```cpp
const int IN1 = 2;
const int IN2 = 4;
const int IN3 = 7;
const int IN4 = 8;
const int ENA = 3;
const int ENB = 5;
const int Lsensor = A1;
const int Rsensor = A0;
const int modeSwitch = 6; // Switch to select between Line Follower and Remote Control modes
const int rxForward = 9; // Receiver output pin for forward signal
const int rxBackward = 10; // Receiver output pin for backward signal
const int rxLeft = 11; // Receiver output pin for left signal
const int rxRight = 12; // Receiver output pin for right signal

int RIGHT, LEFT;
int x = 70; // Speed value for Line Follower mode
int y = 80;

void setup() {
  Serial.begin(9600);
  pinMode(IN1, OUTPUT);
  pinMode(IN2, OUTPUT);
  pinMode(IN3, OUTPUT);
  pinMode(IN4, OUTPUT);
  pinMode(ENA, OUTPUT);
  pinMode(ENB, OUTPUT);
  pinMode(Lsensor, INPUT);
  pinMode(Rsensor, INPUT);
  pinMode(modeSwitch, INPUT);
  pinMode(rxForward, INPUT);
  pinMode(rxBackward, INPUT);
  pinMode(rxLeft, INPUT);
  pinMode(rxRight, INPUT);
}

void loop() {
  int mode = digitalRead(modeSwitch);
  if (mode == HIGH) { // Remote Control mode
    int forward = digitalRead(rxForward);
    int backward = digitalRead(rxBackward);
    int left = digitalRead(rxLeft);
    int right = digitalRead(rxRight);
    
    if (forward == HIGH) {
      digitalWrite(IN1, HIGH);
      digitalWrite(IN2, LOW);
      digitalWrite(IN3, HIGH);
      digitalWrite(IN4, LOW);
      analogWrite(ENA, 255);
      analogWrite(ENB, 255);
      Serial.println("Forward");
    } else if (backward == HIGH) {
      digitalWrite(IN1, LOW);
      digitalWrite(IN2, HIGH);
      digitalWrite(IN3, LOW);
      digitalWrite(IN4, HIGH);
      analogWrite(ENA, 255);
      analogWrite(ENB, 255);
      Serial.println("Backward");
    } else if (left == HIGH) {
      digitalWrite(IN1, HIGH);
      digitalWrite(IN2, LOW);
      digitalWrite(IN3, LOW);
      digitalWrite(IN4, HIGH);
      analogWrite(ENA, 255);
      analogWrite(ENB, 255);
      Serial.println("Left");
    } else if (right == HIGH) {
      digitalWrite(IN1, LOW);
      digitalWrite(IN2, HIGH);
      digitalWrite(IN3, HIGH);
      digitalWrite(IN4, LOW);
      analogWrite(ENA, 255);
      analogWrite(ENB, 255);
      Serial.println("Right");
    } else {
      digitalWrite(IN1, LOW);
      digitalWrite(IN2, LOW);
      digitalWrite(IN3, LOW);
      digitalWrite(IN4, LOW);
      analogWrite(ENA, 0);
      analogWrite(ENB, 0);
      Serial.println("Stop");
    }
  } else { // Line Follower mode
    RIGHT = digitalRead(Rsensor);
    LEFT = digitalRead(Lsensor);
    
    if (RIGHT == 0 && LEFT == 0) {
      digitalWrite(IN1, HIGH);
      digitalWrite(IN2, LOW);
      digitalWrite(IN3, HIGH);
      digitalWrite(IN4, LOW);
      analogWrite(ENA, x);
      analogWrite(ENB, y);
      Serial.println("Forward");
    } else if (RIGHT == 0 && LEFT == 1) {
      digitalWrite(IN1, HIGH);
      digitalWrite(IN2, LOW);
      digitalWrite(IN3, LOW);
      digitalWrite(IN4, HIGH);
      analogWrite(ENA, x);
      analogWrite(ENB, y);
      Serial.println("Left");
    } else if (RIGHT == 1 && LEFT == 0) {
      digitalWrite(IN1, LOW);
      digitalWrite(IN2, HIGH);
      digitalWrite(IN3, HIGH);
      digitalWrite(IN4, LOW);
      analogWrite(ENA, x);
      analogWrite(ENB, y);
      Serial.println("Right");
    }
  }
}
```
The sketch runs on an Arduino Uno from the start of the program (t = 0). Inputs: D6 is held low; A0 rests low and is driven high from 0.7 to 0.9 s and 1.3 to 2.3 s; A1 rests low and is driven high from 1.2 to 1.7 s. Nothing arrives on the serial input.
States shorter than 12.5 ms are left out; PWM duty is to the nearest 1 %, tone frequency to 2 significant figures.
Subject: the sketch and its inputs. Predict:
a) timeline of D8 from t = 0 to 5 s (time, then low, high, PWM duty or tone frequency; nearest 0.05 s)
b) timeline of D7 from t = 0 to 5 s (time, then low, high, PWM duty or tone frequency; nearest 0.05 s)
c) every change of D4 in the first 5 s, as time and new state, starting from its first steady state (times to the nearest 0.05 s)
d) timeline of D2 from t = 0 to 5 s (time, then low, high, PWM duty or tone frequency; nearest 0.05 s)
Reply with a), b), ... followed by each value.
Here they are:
a) 0 s low; 1.2 s high; 1.7 s low
b) 0 s high; 1.2 s low; 1.7 s high
c) 0 s low; 0.7 s high; 0.9 s low; 1.7 s high; 2.3 s low
d) 0 s high; 0.7 s low; 0.9 s high; 1.7 s low; 2.3 s high
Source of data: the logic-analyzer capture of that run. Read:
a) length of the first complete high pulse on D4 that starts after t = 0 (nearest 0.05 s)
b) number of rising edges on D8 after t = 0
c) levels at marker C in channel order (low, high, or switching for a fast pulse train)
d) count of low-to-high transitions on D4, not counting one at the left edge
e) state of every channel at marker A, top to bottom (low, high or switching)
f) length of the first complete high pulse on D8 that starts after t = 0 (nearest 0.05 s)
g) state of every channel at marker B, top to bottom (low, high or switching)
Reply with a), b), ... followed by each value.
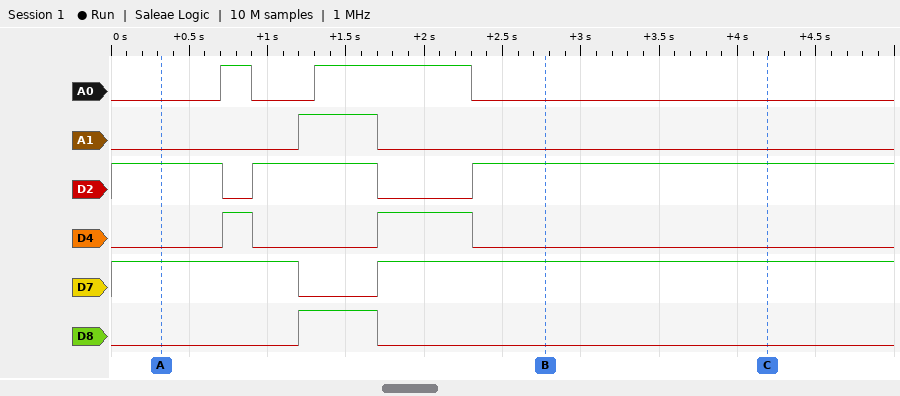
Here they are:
a) 0.20 s
b) 1
c) A0 low, A1 low, D2 high, D4 low, D7 high, D8 low
d) 2
e) A0 low, A1 low, D2 high, D4 low, D7 high, D8 low
f) 0.50 s
g) A0 low, A1 low, D2 high, D4 low, D7 high, D8 low
